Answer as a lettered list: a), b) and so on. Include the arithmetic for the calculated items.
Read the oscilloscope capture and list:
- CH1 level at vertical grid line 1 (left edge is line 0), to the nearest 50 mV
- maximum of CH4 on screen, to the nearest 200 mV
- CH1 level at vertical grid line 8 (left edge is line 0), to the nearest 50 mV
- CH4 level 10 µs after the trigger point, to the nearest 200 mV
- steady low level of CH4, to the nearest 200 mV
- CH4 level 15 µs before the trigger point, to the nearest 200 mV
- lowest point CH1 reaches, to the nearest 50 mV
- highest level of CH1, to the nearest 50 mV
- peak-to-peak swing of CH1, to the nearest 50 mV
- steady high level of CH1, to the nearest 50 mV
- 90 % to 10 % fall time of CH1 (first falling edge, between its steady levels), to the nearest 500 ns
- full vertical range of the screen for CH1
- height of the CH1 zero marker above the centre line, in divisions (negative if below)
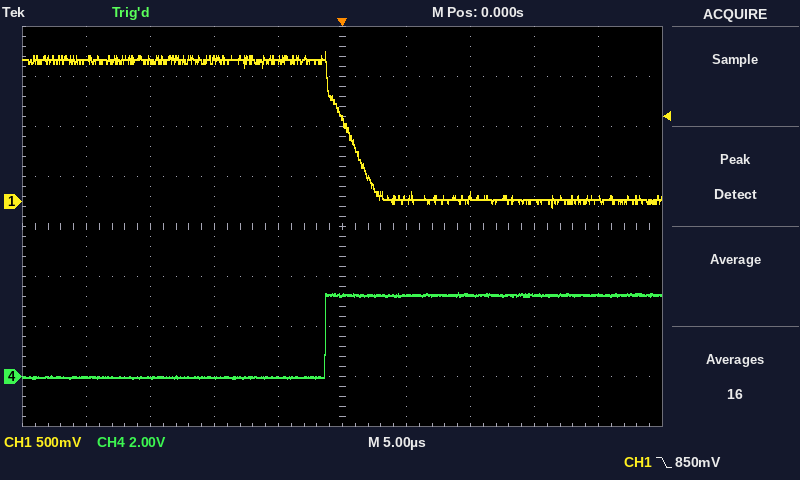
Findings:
a) 1.40 V
b) 3.4 V
c) 0 mV
d) 3.2 V
e) 0.0 V
f) 0.0 V
g) -50 mV
h) 1.50 V
i) 1.50 V − (-50 mV) = 1.55 V
j) 1.40 V
k) 3.5 µs
l) 4 V
m) +0.5 div
